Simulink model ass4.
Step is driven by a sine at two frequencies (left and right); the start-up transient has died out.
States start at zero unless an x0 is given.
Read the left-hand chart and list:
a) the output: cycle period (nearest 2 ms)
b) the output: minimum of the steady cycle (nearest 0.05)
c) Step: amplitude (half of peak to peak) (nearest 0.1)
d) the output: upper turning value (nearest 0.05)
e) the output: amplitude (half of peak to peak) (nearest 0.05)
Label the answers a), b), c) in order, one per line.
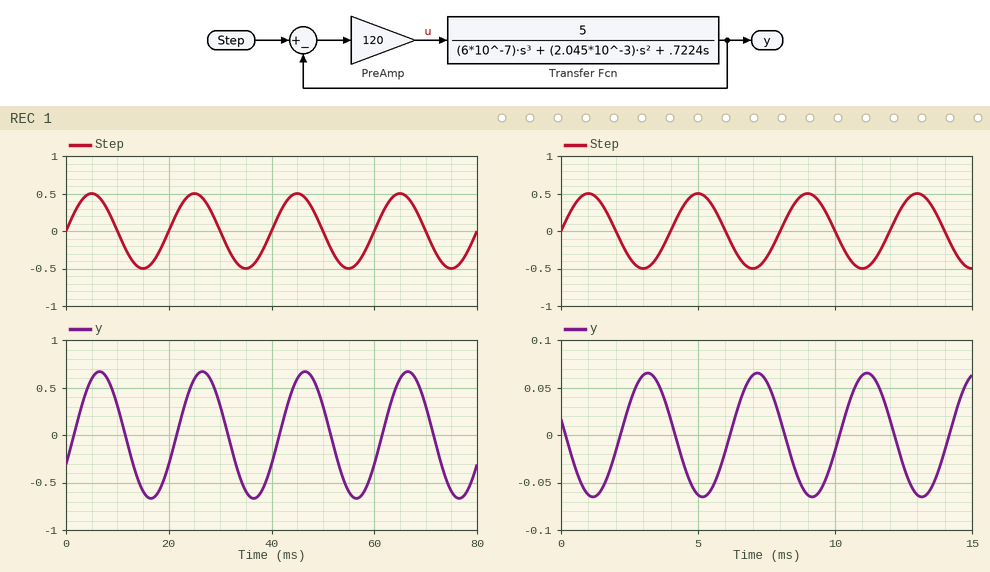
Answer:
a) 20 ms
b) -0.65
c) 0.5
d) 0.65
e) 0.65
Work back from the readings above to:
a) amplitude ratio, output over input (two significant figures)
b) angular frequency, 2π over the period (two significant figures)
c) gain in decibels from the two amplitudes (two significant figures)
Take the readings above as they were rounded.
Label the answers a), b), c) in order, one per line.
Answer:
a) 1.3
b) 0.31 rad/ms
c) 2.3 dB
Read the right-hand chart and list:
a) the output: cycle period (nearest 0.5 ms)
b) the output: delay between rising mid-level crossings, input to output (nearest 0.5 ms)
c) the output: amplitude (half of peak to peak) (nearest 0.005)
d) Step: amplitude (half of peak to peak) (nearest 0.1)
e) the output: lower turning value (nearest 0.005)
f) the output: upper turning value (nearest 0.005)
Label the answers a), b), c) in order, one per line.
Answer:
a) 4.0 ms
b) 2.0 ms
c) 0.065
d) 0.5
e) -0.065
f) 0.065
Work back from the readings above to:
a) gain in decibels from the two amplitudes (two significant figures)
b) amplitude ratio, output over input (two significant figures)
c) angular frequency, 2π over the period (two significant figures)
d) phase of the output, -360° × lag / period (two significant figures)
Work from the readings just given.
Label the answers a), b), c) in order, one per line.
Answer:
a) -18 dB
b) 0.13
c) 1.6 rad/ms
d) -180°
